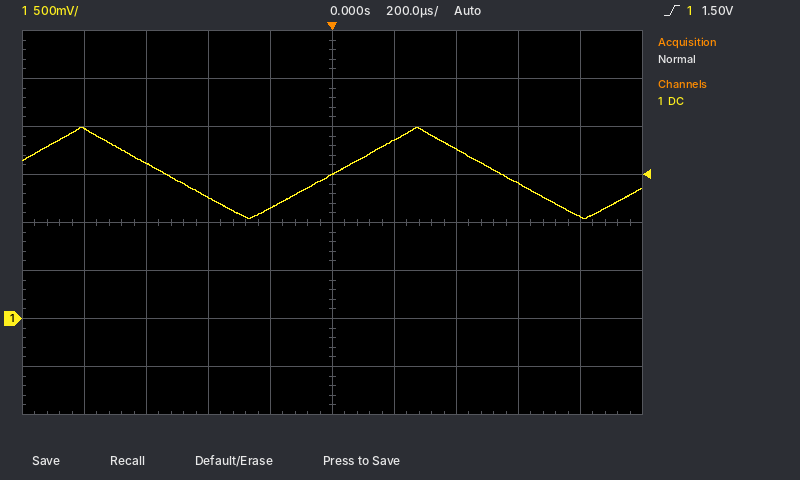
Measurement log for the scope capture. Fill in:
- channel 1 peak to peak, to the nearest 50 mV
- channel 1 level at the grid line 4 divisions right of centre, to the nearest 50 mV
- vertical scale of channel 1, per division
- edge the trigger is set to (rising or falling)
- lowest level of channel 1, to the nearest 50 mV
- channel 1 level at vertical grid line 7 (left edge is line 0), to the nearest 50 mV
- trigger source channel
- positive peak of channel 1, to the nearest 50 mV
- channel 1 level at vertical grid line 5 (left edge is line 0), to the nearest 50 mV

950 mV
1.05 V
500 mV
rising
1.05 V
1.75 V
channel 1
2.00 V
1.50 V
